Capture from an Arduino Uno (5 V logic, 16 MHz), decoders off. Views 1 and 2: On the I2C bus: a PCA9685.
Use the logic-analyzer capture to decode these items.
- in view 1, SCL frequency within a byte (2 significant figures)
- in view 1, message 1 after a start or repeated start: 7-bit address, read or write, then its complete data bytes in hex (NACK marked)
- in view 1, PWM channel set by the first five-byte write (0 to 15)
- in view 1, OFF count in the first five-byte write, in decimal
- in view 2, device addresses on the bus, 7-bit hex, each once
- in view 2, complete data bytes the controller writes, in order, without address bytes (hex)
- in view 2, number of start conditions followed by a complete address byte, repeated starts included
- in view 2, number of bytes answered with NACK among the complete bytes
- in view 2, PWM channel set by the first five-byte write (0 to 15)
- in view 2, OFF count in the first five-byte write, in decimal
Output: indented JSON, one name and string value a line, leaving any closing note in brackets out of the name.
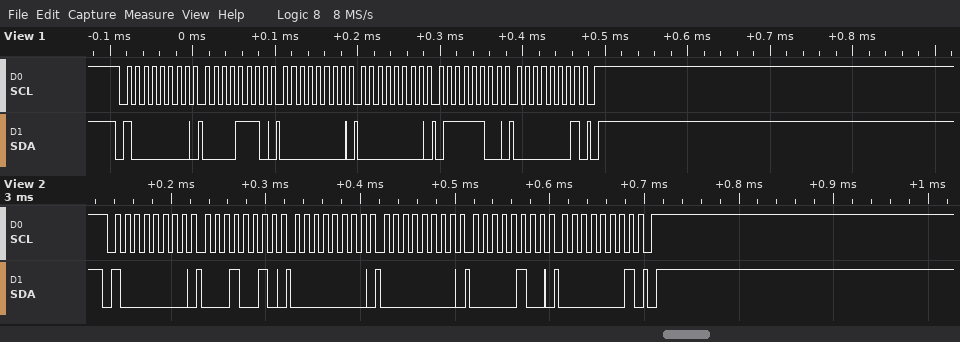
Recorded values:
{
  "in view 1, SCL frequency within a byte": "100 kHz",
  "in view 1, message 1 after a start or repeated start: 7-bit address, read or write, then its complete data bytes in hex": "0x40 write: 0E 00 00 7C 01",
  "in view 1, PWM channel set by the first five-byte write": "2",
  "in view 1, OFF count in the first five-byte write, in decimal": "380",
  "in view 2, device addresses on the bus, 7-bit hex, each once": "0x40",
  "in view 2, complete data bytes the controller writes, in order, without address bytes": "12 00 00 04 01",
  "in view 2, number of start conditions followed by a complete address byte, repeated starts included": "1",
  "in view 2, number of bytes answered with NACK among the complete bytes": "0",
  "in view 2, PWM channel set by the first five-byte write": "3",
  "in view 2, OFF count in the first five-byte write, in decimal": "260"
}
